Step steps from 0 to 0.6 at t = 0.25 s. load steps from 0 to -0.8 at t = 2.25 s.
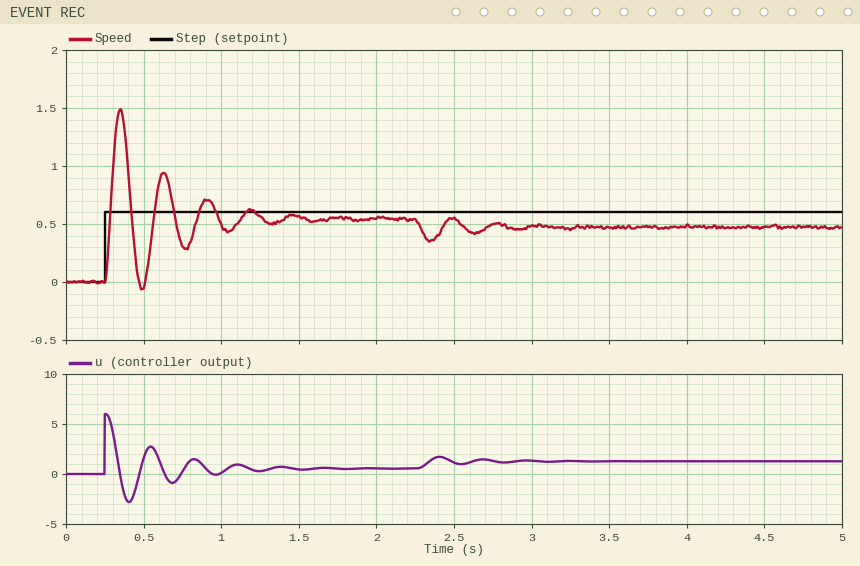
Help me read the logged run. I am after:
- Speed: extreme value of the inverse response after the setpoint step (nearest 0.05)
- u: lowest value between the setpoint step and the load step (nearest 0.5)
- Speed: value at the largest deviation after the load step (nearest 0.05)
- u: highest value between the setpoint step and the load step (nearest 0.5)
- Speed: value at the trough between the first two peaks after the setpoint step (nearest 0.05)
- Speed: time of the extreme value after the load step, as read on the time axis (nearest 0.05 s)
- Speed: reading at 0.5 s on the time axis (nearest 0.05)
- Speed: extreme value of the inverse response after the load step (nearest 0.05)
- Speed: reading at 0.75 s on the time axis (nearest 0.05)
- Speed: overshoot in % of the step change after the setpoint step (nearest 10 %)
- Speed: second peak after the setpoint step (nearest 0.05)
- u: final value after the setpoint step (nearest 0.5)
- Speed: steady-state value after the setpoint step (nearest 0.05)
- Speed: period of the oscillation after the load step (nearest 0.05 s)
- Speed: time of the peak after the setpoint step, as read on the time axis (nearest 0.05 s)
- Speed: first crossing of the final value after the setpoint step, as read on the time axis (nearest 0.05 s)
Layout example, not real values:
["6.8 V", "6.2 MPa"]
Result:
["-0.05", "-3.0", "0.35", "6.0", "-0.05", "2.35 s", "-0.05", "0.55", "0.30", "170 %", "0.95", "0.5", "0.55", "0.30 s", "0.35 s", "0.30 s"]
